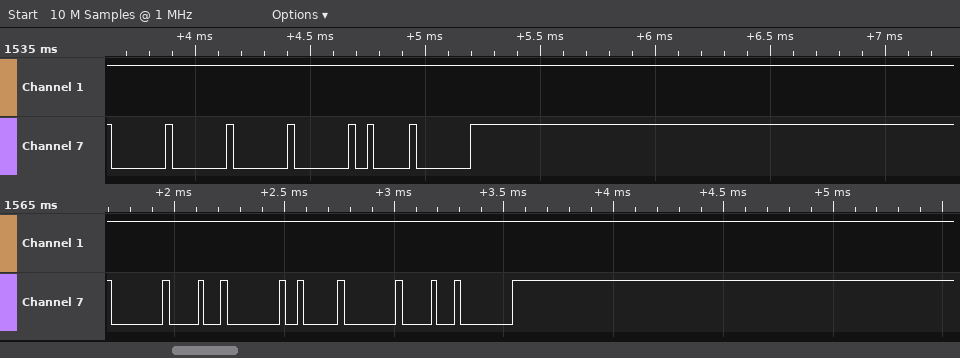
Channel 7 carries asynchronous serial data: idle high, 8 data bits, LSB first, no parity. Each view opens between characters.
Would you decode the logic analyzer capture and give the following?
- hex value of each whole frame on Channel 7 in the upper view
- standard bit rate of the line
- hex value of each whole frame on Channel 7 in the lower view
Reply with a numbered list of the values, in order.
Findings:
1. 00, 00, 00, 00, 02, 00
2. 38400 baud
3. 00, 10, 00, 02, 00, 10, 00
